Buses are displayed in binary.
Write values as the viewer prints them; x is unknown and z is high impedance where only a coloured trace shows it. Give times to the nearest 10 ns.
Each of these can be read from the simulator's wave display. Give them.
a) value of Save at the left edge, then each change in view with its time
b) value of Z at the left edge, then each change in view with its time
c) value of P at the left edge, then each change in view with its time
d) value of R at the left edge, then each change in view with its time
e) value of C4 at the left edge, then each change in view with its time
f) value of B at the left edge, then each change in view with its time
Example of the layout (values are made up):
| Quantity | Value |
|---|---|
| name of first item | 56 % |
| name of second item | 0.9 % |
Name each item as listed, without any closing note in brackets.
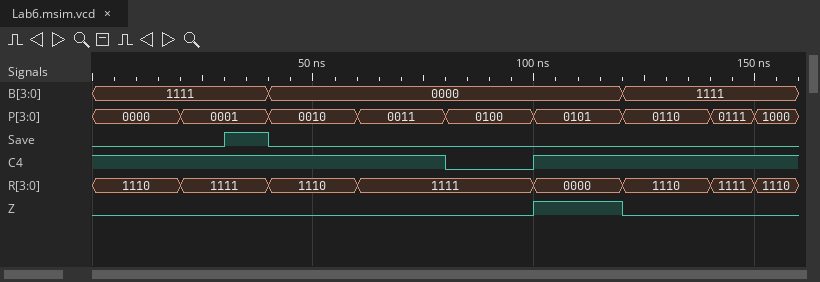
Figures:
| Quantity | Value |
|---|---|
| value of Save at the left edge, then each change in view with its time | 0, 1 at 30 ns, 0 at 40 ns |
| value of Z at the left edge, then each change in view with its time | 0, 1 at 100 ns, 0 at 120 ns |
| value of P at the left edge, then each change in view with its time | 0000, 0001 at 20 ns, 0010 at 40 ns, 0011 at 60 ns, 0100 at 80 ns, 0101 at 100 ns, 0110 at 120 ns, 0111 at 140 ns, 1000 at 150 ns |
| value of R at the left edge, then each change in view with its time | 1110, 1111 at 20 ns, 1110 at 40 ns, 1111 at 60 ns, 0000 at 100 ns, 1110 at 120 ns, 1111 at 140 ns, 1110 at 150 ns |
| value of C4 at the left edge, then each change in view with its time | 1, 0 at 80 ns, 1 at 100 ns |
| value of B at the left edge, then each change in view with its time | 1111, 0000 at 40 ns, 1111 at 120 ns |
